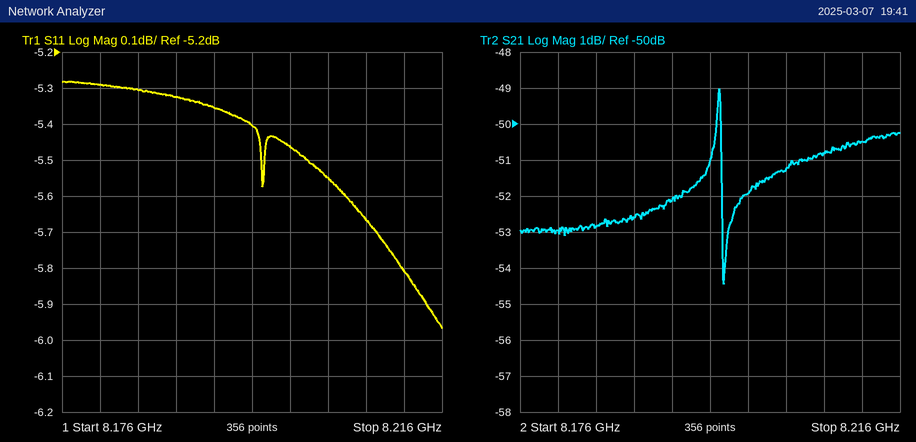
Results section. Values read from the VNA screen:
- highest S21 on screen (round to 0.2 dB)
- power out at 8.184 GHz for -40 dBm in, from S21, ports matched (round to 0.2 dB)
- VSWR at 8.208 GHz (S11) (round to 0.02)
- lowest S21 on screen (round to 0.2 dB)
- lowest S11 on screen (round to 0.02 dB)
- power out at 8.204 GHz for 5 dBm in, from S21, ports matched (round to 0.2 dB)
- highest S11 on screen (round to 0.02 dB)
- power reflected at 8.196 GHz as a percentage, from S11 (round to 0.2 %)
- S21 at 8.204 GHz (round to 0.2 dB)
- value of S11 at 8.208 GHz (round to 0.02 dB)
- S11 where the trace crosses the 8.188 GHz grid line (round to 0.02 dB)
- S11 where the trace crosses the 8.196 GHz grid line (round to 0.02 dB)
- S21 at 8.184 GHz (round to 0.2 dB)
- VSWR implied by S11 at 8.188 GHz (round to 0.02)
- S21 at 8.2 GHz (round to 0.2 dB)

-49.0 dB
-92.8 dBm
3.18
-54.4 dB
-5.96 dB
-46.2 dBm
-5.28 dB
28.8 %
-51.2 dB
-5.66 dB
-5.32 dB
-5.40 dB
-52.8 dB
3.36
-52.0 dB
